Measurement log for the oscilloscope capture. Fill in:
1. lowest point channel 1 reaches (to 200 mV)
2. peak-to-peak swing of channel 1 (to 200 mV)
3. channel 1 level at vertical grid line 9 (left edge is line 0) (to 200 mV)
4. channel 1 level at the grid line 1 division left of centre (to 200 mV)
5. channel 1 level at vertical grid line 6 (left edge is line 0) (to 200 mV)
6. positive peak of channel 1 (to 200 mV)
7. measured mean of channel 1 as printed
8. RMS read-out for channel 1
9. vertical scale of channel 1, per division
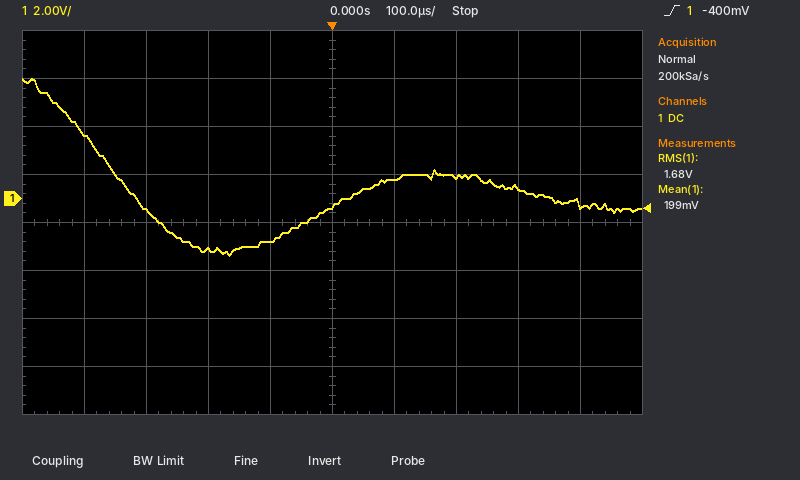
-2.4 V
7.4 V
-200 mV
-1.8 V
800 mV
5.0 V
199 mV
1.68 V
2 V
